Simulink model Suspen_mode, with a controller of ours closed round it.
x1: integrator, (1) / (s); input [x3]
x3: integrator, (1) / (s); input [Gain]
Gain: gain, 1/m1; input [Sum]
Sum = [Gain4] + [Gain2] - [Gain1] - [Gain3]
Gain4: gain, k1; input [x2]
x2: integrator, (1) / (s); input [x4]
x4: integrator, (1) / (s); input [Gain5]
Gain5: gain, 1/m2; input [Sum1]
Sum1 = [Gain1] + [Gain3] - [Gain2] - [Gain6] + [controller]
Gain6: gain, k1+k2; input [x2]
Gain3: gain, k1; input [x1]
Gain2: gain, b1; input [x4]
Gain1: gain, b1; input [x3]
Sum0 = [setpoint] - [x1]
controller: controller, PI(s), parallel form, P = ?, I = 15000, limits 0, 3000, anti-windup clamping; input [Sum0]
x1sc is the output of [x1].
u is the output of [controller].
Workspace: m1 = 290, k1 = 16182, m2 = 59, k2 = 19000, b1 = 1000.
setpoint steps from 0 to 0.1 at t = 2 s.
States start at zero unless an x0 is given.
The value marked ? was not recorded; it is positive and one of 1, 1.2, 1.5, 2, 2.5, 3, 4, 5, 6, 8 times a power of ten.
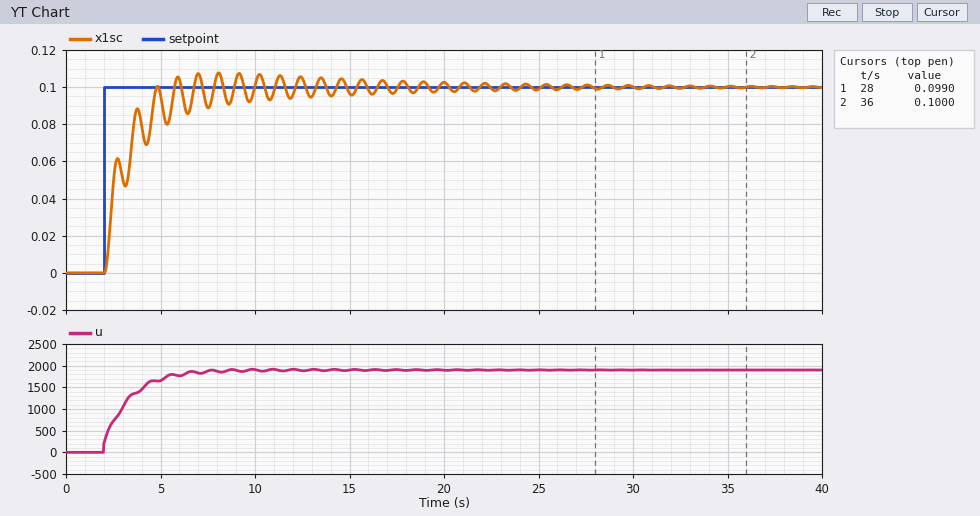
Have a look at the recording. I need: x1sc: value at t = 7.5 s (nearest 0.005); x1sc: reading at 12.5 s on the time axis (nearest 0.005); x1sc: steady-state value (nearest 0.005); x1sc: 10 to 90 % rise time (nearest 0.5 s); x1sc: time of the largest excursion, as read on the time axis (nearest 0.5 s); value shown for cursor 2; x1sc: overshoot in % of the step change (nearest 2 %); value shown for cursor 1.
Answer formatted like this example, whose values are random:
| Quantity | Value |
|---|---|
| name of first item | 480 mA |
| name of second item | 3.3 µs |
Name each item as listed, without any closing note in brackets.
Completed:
| Quantity | Value |
|---|---|
| x1sc: value at t = 7.5 s | 0.090 |
| x1sc: reading at 12.5 s on the time axis | 0.105 |
| x1sc: steady-state value | 0.100 |
| x1sc: 10 to 90 % rise time | 2.5 s |
| x1sc: time of the largest excursion, as read on the time axis | 8.0 s |
| value shown for cursor 2 | 0.1000 |
| x1sc: overshoot in % of the step change | 8 % |
| value shown for cursor 1 | 0.0990 |
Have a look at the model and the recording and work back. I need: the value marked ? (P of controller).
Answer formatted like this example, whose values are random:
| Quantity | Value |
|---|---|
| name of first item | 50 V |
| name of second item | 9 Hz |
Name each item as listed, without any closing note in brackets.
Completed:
| Quantity | Value |
|---|---|
| the value marked ? | 2000 |
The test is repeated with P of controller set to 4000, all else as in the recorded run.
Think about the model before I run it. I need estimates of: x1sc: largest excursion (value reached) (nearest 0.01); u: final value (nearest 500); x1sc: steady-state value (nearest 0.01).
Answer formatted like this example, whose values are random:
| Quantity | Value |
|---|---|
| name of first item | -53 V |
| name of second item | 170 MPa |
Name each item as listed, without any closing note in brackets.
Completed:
| Quantity | Value |
|---|---|
| x1sc: largest excursion (value reached) | 0.11 |
| u: final value | 2000 |
| x1sc: steady-state value | 0.10 |
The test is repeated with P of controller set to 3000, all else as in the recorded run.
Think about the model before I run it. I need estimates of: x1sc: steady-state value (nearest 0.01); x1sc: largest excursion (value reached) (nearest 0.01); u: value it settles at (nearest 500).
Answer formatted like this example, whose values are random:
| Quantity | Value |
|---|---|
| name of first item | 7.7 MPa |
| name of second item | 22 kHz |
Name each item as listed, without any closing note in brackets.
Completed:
| Quantity | Value |
|---|---|
| x1sc: steady-state value | 0.10 |
| x1sc: largest excursion (value reached) | 0.11 |
| u: value it settles at | 2000 |
